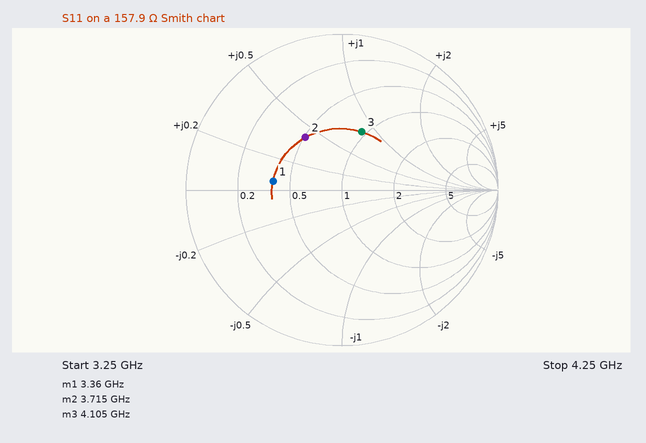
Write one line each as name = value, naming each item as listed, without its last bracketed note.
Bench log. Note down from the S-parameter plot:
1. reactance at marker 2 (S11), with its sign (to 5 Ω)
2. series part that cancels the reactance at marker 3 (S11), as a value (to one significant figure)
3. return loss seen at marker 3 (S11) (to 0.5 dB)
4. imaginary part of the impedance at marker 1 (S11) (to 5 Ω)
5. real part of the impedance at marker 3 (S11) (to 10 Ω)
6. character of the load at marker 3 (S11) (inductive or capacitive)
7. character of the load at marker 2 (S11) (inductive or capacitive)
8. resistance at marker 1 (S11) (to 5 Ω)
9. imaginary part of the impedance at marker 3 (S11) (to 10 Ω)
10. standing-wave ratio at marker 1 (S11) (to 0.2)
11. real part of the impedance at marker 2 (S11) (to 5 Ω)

reactance at marker 2 (S11), with its sign = +65 Ω
series part that cancels the reactance at marker 3 (S11), as a value = 300 fF
return loss seen at marker 3 (S11) = 8.0 dB
imaginary part of the impedance at marker 1 (S11) = +10 Ω
real part of the impedance at marker 3 (S11) = 150 Ω
character of the load at marker 3 (S11) = inductive
character of the load at marker 2 (S11) = inductive
resistance at marker 1 (S11) = 60 Ω
imaginary part of the impedance at marker 3 (S11) = +130 Ω
standing-wave ratio at marker 1 (S11) = 2.6
real part of the impedance at marker 2 (S11) = 80 Ω
